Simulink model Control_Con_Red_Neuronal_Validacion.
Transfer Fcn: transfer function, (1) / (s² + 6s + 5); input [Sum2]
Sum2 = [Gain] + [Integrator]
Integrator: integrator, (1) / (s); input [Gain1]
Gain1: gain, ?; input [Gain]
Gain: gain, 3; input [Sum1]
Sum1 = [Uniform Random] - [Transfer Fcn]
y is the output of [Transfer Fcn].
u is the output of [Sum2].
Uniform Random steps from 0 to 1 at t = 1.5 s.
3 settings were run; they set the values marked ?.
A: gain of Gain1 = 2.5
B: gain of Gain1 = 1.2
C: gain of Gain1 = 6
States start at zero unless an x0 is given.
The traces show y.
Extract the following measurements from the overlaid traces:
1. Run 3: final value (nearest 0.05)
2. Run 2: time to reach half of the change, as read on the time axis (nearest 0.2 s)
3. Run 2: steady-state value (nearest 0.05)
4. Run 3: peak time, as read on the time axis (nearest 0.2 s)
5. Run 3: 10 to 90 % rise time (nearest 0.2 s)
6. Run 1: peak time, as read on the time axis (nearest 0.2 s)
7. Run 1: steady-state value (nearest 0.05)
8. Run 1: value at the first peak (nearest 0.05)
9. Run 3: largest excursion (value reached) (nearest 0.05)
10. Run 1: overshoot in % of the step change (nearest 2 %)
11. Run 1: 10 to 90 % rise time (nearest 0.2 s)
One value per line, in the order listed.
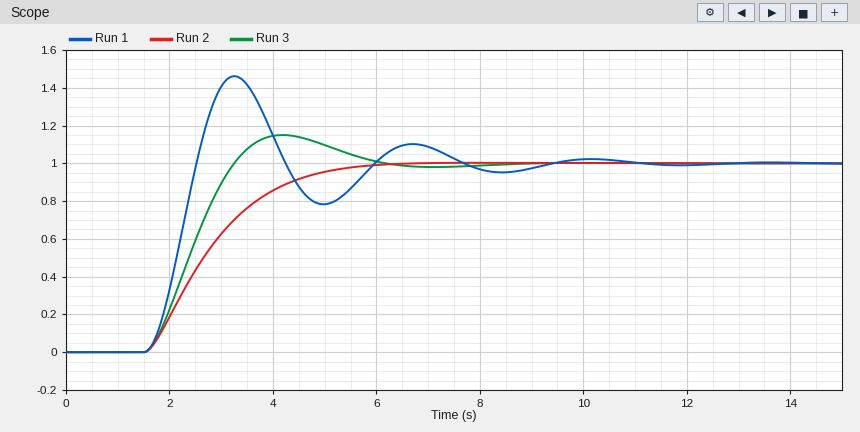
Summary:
1.00
2.6 s
1.00
4.2 s
1.2 s
3.2 s
1.00
1.45
1.15
46 %
0.6 s
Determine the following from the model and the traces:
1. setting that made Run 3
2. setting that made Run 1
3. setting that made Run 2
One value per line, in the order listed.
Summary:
A
C
B
